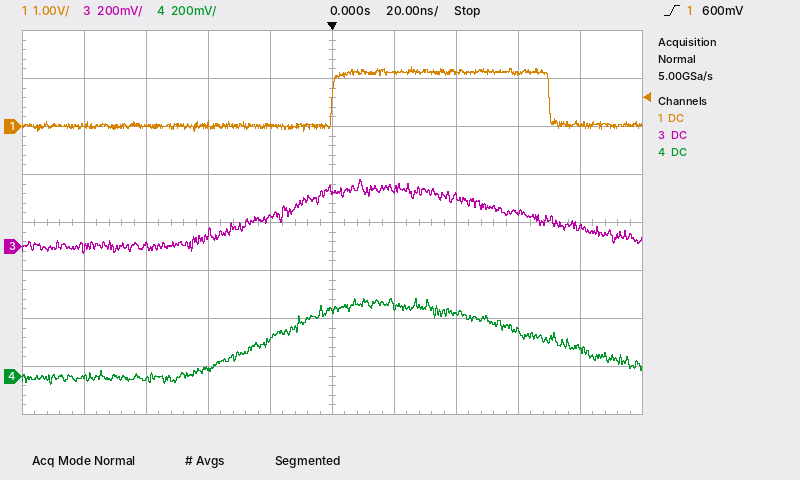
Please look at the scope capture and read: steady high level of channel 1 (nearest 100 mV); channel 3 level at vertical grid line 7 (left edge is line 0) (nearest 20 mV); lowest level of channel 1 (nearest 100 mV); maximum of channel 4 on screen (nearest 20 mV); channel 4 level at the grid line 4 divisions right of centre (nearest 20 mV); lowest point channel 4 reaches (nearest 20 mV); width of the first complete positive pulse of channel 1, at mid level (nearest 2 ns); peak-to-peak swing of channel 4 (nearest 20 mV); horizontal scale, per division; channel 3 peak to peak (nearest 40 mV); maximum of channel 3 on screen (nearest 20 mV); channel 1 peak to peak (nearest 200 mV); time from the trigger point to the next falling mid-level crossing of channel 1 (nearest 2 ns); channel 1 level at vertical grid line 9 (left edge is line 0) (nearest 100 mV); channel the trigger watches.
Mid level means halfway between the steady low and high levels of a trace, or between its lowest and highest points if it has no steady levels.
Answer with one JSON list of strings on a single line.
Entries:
["1.1 V", "200 mV", "-100 mV", "320 mV", "120 mV", "-40 mV", "70 ns", "360 mV", "20 ns", "320 mV", "280 mV", "1.4 V", "70 ns", "0.0 V", "channel 1"]
